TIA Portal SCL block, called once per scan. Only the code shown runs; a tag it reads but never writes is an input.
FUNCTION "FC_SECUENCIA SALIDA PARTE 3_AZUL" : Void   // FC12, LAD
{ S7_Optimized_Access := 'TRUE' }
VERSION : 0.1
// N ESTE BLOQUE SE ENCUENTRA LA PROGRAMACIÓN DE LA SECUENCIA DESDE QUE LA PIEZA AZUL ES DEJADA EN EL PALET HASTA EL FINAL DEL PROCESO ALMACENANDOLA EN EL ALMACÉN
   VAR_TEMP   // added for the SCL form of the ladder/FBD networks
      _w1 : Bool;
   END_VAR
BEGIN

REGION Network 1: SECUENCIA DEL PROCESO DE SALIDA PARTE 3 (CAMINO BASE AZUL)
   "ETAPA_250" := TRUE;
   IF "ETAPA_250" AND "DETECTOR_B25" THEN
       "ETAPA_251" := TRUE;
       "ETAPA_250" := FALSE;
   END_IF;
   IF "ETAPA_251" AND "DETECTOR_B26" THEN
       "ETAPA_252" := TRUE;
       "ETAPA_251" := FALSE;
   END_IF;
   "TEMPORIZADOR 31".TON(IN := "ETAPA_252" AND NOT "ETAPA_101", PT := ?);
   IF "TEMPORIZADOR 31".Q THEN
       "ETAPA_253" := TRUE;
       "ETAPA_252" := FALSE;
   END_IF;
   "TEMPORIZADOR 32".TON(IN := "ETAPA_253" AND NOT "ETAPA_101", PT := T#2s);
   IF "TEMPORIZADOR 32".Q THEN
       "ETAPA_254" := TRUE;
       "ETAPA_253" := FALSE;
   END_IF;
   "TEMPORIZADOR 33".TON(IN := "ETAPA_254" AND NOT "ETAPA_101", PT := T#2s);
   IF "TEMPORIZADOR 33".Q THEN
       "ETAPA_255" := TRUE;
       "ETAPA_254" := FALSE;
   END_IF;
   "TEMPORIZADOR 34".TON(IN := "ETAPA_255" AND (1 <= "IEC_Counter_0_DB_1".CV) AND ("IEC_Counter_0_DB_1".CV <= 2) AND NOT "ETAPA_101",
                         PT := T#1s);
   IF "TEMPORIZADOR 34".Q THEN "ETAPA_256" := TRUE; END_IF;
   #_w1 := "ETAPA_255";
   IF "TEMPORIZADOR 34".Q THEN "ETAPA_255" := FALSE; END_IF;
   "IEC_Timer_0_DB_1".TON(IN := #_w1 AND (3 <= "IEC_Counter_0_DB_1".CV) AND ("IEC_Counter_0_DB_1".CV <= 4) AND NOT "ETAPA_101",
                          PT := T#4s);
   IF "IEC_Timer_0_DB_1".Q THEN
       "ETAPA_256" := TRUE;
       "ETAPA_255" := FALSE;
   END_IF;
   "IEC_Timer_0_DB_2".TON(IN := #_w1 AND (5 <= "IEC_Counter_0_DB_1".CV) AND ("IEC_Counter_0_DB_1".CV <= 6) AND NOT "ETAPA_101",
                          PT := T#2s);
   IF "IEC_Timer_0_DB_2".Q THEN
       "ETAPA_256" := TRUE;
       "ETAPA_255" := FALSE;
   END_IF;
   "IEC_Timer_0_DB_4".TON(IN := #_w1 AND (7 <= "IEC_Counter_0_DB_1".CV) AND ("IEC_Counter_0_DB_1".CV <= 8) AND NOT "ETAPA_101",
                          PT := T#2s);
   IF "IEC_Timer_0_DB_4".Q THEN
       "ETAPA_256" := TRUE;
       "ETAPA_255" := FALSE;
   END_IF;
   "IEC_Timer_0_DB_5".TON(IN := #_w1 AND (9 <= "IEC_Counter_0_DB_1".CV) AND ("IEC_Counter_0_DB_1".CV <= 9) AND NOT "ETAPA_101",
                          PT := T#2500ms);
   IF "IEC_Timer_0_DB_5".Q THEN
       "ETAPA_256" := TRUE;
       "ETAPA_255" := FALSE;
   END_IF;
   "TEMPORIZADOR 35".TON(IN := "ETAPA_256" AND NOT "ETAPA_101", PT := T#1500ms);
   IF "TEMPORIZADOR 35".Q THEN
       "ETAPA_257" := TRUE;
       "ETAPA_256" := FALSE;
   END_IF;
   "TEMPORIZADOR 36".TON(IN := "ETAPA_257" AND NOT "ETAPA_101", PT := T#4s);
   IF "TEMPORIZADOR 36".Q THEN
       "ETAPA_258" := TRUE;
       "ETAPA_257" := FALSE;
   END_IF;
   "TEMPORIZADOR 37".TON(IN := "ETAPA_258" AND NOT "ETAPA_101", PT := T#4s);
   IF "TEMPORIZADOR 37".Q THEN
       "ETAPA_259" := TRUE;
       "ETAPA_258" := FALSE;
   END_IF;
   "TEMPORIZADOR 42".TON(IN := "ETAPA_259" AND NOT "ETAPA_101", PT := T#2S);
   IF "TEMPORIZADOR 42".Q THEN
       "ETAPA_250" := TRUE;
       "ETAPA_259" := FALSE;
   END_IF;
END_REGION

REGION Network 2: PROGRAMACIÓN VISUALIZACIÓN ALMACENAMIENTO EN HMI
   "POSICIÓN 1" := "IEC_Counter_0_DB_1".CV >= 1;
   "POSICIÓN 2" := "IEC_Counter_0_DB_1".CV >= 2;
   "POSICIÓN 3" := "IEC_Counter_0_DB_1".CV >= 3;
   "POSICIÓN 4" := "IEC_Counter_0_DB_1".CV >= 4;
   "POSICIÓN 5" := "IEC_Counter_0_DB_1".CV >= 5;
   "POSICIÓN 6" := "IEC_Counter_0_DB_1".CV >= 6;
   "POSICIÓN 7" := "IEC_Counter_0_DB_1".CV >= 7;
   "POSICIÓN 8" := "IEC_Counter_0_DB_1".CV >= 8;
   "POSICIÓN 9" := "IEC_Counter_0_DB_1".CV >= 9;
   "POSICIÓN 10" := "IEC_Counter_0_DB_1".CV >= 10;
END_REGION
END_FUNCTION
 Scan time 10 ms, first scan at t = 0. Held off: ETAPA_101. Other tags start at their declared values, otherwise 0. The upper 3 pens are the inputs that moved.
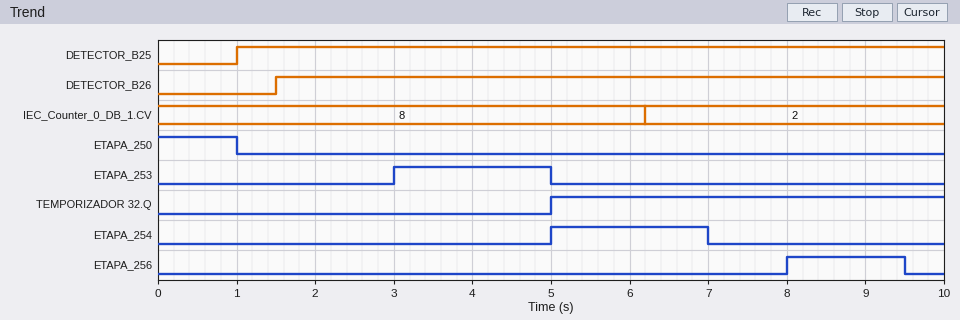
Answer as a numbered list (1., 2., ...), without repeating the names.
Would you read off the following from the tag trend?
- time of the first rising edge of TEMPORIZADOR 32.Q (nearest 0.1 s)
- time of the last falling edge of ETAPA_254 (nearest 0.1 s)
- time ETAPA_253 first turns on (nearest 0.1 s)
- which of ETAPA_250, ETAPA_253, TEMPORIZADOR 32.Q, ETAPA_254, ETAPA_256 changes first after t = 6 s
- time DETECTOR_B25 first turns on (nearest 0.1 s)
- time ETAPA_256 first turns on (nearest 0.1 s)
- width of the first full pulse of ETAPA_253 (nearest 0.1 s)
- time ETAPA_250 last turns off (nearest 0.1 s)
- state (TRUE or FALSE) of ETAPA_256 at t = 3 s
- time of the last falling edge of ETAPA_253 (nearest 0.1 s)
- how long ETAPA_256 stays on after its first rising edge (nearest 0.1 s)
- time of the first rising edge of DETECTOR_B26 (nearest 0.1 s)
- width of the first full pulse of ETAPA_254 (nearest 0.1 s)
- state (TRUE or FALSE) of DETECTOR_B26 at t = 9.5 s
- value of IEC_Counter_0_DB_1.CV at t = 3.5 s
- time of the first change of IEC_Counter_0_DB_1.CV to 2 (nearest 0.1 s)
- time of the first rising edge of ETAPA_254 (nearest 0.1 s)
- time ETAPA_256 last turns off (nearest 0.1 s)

1. 5.0 s
2. 7.0 s
3. 3.0 s
4. ETAPA_254
5. 1.0 s
6. 8.0 s
7. 2.0 s
8. 1.0 s
9. FALSE
10. 5.0 s
11. 1.5 s
12. 1.5 s
13. 2.0 s
14. TRUE
15. 8
16. 6.2 s
17. 5.0 s
18. 9.5 s
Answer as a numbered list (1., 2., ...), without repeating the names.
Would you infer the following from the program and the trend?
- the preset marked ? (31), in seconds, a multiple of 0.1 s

1. 1.5 s
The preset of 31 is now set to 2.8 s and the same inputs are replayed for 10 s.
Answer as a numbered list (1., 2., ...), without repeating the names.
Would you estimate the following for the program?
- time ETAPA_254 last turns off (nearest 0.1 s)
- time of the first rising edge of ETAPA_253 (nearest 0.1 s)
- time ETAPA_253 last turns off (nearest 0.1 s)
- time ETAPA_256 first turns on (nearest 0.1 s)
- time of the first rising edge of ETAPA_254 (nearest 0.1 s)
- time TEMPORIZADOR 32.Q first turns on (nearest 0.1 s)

1. 8.3 s
2. 4.3 s
3. 6.3 s
4. 9.3 s
5. 6.3 s
6. 6.3 s
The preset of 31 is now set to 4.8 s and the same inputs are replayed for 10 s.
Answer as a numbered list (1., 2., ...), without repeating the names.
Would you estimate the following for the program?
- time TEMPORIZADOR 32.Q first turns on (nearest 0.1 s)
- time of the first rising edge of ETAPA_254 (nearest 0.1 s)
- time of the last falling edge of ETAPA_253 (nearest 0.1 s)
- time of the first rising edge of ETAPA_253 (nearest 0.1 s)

1. 8.3 s
2. 8.3 s
3. 8.3 s
4. 6.3 s
